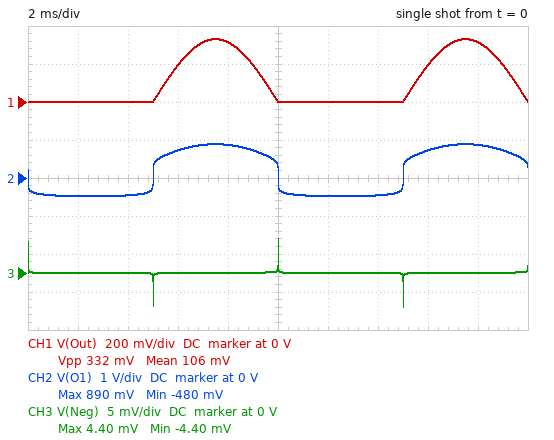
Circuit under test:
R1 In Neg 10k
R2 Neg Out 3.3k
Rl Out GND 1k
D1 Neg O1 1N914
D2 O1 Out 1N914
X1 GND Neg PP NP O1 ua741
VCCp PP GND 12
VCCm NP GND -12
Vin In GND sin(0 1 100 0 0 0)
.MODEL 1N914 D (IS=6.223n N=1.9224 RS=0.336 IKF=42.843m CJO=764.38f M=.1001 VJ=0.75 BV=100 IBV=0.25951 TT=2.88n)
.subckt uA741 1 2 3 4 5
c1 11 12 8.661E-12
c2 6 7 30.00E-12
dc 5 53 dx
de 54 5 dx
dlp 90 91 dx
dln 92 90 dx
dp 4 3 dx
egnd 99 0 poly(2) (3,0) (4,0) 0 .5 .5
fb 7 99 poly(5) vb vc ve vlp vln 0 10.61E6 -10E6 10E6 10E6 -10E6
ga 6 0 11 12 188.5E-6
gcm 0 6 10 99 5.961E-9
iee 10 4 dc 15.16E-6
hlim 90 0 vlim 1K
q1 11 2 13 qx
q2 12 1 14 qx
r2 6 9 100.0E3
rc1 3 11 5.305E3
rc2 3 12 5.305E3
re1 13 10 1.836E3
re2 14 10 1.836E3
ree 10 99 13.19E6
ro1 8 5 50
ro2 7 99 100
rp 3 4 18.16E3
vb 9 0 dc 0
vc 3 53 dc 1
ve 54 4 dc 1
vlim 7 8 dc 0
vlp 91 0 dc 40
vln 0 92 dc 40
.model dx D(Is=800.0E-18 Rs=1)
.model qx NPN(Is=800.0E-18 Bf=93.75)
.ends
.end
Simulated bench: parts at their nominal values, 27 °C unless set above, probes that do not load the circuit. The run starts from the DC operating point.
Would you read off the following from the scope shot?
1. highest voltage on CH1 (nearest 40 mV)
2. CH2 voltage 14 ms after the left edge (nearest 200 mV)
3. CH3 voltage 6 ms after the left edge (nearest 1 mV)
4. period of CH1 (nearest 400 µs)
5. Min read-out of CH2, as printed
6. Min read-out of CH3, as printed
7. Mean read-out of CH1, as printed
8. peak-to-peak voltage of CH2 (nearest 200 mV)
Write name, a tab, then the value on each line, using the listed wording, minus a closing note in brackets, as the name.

highest voltage on CH1	320 mV
CH2 voltage 14 ms after the left edge	-400 mV
CH3 voltage 6 ms after the left edge	0 V
period of CH1	10.0 ms
Min read-out of CH2, as printed	-480 mV
Min read-out of CH3, as printed	-4.40 mV
Mean read-out of CH1, as printed	106 mV
peak-to-peak voltage of CH2	1.4 V
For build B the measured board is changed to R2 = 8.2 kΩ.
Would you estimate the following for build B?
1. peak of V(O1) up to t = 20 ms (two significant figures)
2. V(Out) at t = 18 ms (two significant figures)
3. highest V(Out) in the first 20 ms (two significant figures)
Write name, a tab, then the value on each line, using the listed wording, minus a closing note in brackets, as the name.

peak of V(O1) up to t = 20 ms	1.4 V
V(Out) at t = 18 ms	780 mV
highest V(Out) in the first 20 ms	820 mV
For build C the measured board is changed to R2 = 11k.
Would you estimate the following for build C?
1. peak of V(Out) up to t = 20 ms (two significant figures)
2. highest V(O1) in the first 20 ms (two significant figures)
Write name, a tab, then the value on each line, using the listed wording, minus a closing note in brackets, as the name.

peak of V(Out) up to t = 20 ms	1.1 V
highest V(O1) in the first 20 ms	1.7 V
